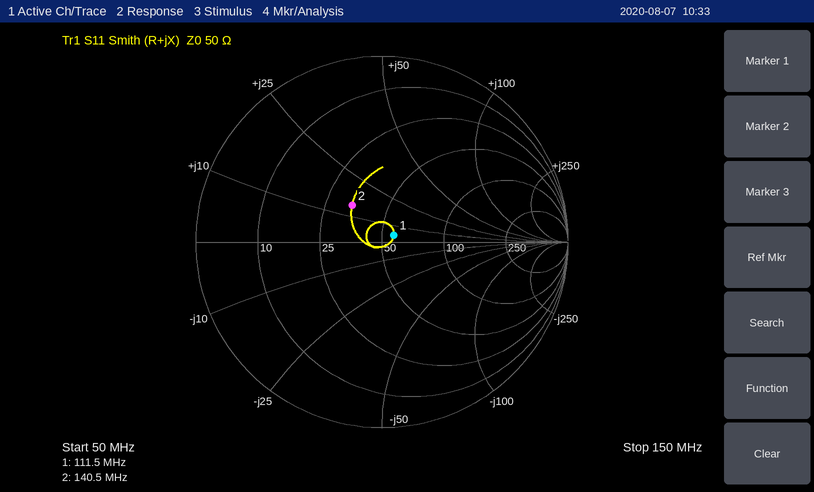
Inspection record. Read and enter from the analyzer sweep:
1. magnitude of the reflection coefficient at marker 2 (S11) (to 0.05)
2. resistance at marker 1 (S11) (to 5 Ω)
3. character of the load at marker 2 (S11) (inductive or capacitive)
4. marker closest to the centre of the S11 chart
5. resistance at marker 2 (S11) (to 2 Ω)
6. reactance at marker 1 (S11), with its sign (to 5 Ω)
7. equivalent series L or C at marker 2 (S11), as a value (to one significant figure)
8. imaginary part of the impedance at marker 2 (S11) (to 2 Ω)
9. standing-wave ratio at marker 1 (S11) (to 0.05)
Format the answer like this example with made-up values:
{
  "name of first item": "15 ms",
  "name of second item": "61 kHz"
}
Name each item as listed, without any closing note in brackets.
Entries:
{
  "magnitude of the reflection coefficient at marker 2 (S11)": "0.25",
  "resistance at marker 1 (S11)": "55 Ω",
  "character of the load at marker 2 (S11)": "inductive",
  "marker closest to the centre of the S11 chart": "marker 1",
  "resistance at marker 2 (S11)": "34 Ω",
  "reactance at marker 1 (S11), with its sign": "+5 Ω",
  "equivalent series L or C at marker 2 (S11), as a value": "20 nH",
  "imaginary part of the impedance at marker 2 (S11)": "+14 Ω",
  "standing-wave ratio at marker 1 (S11)": "1.15"
}
